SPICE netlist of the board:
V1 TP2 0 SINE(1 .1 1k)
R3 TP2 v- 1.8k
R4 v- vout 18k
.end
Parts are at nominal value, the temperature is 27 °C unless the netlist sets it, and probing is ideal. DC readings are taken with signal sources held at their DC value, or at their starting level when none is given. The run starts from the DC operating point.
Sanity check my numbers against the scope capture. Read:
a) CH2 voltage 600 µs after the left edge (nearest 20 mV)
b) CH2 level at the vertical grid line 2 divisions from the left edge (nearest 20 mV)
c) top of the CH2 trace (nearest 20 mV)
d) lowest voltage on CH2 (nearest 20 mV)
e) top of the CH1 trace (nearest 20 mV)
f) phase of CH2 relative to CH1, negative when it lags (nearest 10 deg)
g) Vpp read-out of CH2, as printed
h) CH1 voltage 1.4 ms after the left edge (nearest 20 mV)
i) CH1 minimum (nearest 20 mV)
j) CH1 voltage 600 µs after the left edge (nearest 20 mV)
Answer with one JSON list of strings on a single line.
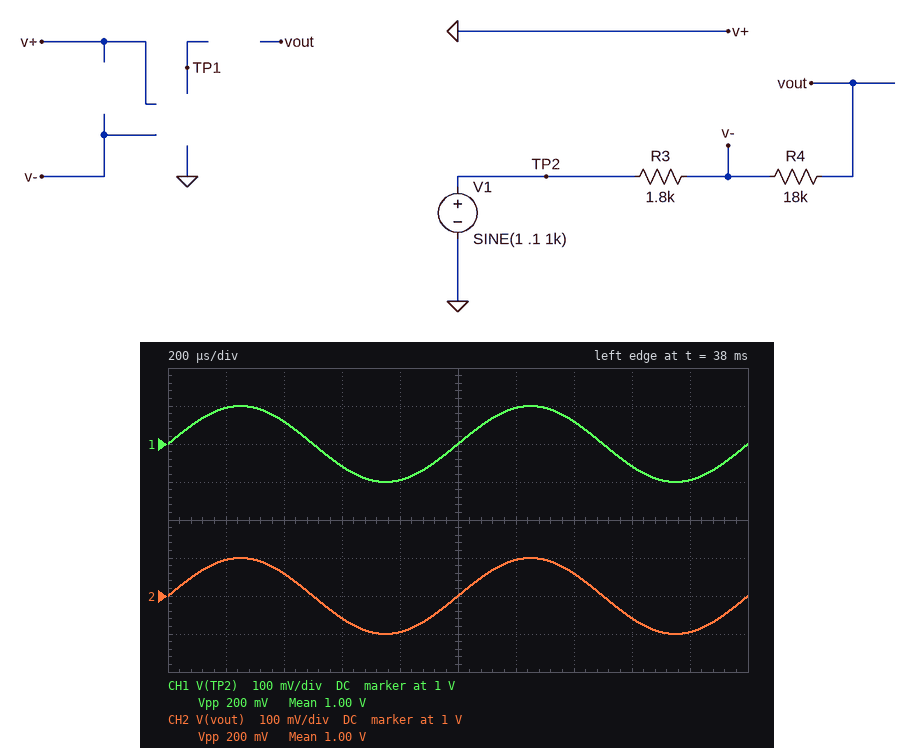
["940 mV", "1.06 V", "1.10 V", "900 mV", "1.10 V", "0 deg", "200 mV", "1.06 V", "900 mV", "940 mV"]
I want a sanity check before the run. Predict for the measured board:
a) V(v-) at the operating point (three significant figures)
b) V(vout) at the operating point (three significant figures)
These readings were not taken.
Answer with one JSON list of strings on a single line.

["1.00 V", "1.00 V"]
